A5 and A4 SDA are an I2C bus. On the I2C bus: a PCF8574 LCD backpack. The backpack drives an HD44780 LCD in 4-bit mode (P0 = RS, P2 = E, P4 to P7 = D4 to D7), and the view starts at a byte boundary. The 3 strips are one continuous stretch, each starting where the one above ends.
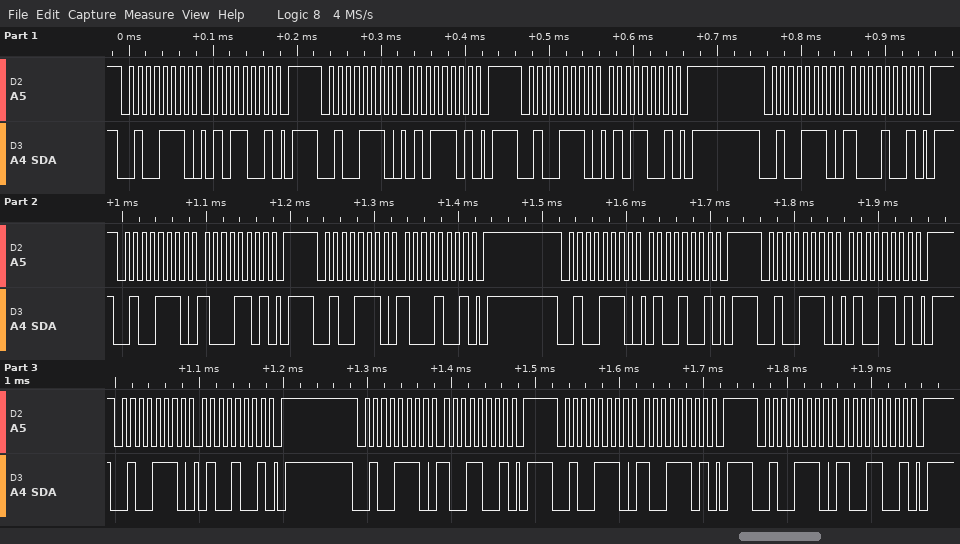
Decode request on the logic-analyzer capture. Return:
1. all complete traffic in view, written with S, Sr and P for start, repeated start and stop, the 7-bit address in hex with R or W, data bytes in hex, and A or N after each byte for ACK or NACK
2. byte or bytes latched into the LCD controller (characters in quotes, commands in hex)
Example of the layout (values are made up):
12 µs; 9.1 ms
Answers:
S 27W A 59 A P S 27W A 5D A P S 27W A 59 A P S 27W A 89 A P S 27W A 8D A P S 27W A 89 A P S 27W A 49 A P S 27W A 4D A P S 27W A 49 A P S 27W A 99 A P S 27W A 9D A P S 27W A 99 A P; 'X' 'I'
